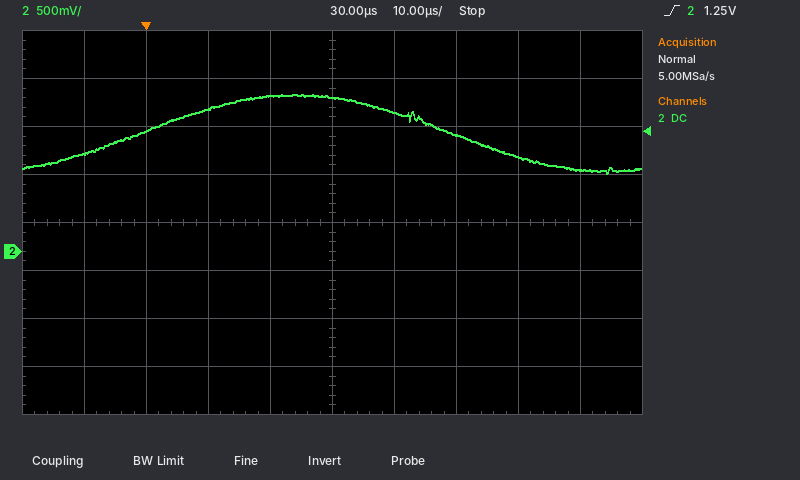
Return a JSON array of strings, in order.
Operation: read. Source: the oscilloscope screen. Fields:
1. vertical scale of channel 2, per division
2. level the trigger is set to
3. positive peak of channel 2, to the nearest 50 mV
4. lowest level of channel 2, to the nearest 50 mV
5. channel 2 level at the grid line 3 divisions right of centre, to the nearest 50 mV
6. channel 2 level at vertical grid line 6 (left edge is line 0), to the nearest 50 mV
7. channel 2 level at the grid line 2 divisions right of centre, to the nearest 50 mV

["500 mV", "1.25 V", "1.65 V", "800 mV", "1.00 V", "1.45 V", "1.20 V"]
